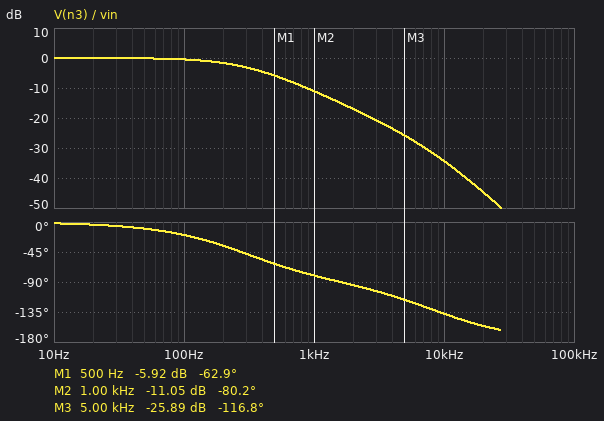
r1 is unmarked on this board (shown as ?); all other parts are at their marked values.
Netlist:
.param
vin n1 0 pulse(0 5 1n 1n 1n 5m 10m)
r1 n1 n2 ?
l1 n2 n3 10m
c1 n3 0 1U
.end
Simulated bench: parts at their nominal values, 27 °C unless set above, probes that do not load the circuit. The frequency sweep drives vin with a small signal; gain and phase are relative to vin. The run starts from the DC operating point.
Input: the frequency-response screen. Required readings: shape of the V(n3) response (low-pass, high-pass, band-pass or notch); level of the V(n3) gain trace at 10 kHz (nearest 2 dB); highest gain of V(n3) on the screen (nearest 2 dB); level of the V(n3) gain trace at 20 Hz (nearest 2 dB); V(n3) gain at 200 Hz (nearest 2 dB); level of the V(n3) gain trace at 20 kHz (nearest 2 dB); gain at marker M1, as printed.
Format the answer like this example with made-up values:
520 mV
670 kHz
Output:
low-pass
-34 dB
0 dB
0 dB
-2 dB
-44 dB
-5.92 dB
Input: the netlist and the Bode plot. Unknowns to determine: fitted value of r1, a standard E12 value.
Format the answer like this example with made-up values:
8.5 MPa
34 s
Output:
560 Ω
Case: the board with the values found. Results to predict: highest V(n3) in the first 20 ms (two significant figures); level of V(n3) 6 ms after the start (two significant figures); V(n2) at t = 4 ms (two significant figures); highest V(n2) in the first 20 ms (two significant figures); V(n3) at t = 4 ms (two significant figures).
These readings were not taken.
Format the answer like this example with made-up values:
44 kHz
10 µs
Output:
5.0 V
820 mV
5.0 V
5.0 V
5.0 V
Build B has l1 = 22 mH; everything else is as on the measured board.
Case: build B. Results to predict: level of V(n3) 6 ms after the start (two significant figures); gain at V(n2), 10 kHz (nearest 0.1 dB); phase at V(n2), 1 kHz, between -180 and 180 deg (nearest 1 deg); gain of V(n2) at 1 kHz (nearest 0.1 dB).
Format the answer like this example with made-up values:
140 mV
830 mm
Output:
790 mV
-0.7 dB
-88 deg
-28.6 dB
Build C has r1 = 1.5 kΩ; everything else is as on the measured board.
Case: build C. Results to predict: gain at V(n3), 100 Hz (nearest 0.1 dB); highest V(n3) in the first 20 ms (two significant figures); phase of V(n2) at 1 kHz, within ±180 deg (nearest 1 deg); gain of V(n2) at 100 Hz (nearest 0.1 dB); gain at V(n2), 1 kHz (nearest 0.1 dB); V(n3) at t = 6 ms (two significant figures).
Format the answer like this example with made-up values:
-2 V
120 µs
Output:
-2.7 dB
4.8 V
-86 deg
-2.8 dB
-23.9 dB
2.5 V
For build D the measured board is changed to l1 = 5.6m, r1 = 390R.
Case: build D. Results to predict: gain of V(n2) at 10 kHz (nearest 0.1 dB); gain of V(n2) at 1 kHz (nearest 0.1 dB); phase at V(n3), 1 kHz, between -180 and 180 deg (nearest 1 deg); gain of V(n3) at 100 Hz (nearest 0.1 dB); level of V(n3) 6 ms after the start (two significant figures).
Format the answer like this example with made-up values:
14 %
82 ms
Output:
-3.7 dB
-10.4 dB
-72 deg
-0.2 dB
360 mV
